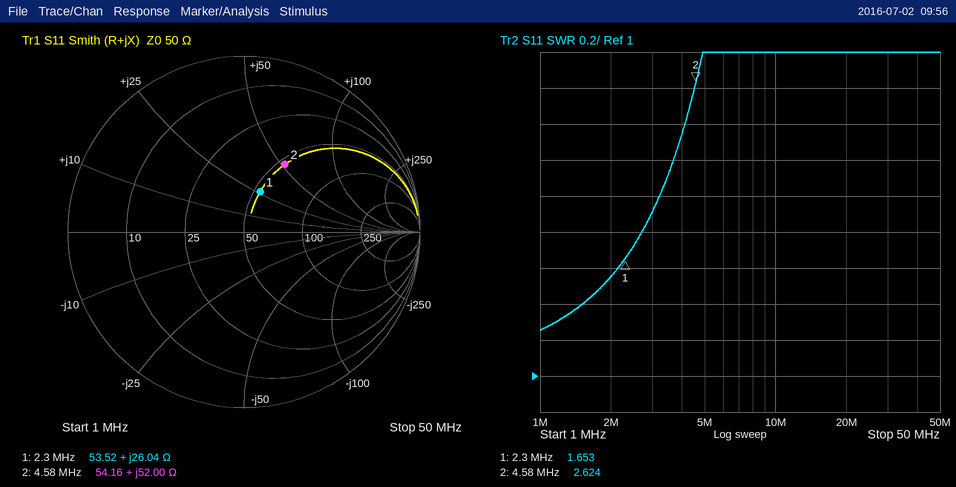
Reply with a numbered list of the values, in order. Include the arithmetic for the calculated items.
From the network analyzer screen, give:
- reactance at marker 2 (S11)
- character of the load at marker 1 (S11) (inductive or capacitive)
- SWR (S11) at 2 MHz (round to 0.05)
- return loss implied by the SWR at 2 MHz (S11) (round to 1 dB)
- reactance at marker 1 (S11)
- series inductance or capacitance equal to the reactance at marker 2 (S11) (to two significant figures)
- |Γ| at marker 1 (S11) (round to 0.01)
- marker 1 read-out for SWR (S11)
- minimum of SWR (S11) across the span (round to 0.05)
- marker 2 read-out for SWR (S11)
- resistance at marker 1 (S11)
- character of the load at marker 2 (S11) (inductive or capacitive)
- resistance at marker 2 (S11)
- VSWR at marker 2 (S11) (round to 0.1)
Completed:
1. +52.00 Ω
2. inductive
3. 1.55
4. −20 log10((1.55 − 1)/(1.55 + 1)) ≈ 13 dB
5. +26.04 Ω
6. L = 52 Ω/(2π × 4.58 MHz) ≈ 1.8 µH
7. 0.25
8. 1.653
9. 1.25
10. 2.624
11. 53.52 Ω
12. inductive
13. 54.16 Ω
14. 2.6
